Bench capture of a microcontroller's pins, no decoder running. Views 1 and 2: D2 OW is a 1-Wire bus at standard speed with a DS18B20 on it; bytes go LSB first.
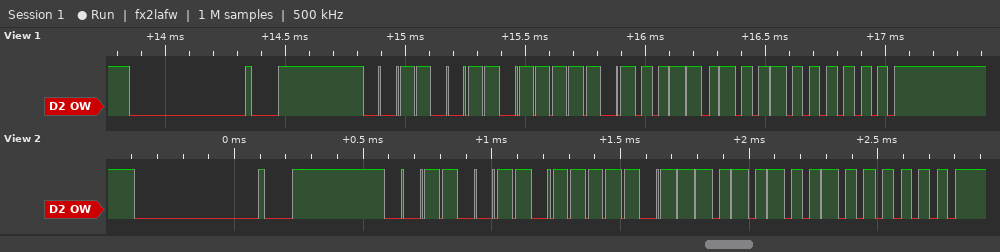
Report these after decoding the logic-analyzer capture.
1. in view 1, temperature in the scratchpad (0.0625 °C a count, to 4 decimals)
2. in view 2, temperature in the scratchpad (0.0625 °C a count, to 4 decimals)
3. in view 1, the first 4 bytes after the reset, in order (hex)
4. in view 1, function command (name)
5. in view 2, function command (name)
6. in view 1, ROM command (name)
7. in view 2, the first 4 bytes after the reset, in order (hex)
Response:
18.7500 °C
18.6875 °C
CC BE 2C 01
Read Scratchpad
Read Scratchpad
Skip ROM
CC BE 2B 01
